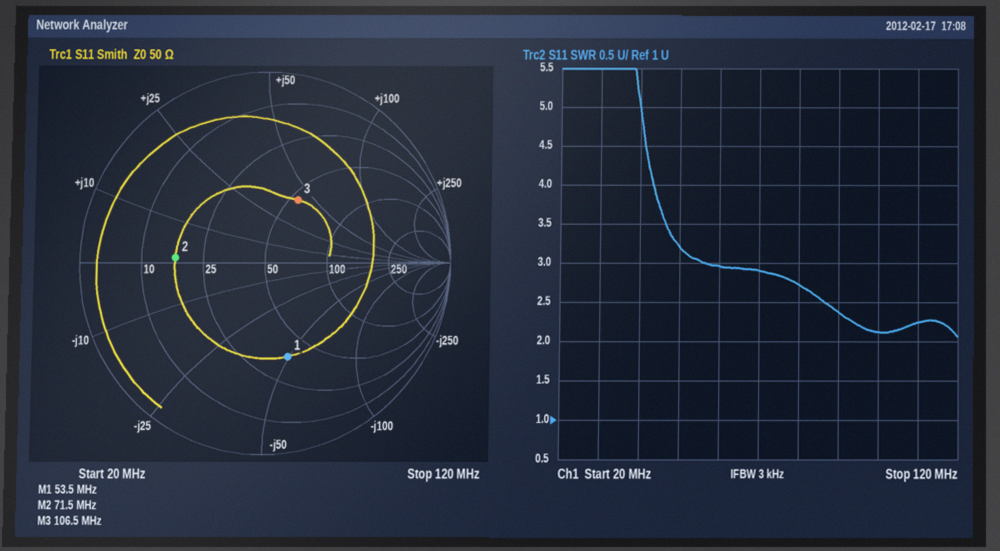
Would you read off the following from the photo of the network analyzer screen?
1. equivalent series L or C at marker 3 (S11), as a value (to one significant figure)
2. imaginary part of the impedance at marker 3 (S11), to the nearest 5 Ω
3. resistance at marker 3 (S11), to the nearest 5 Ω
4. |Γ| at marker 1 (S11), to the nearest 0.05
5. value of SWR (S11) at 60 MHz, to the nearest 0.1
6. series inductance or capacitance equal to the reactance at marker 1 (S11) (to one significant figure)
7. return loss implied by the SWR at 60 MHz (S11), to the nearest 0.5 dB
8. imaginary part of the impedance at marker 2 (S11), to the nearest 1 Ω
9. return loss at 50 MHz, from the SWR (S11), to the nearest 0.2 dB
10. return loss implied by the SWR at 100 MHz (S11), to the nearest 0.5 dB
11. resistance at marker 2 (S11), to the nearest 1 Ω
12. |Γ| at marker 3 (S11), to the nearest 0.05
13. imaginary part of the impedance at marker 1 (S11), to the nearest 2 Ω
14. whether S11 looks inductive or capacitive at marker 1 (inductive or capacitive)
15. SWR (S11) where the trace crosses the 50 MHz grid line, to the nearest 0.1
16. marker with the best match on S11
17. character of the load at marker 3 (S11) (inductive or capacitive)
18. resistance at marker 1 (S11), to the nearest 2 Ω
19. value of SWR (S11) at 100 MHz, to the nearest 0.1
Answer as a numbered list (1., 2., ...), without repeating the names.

1. 60 nH
2. +40 Ω
3. 55 Ω
4. 0.50
5. 3.0
6. 60 pF
7. 6.0 dB
8. +1 Ω
9. 5.6 dB
10. 9.0 dB
11. 17 Ω
12. 0.35
13. -50 Ω
14. capacitive
15. 3.2
16. marker 3
17. inductive
18. 38 Ω
19. 2.1
